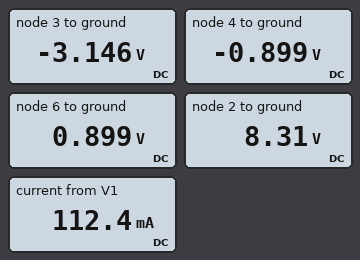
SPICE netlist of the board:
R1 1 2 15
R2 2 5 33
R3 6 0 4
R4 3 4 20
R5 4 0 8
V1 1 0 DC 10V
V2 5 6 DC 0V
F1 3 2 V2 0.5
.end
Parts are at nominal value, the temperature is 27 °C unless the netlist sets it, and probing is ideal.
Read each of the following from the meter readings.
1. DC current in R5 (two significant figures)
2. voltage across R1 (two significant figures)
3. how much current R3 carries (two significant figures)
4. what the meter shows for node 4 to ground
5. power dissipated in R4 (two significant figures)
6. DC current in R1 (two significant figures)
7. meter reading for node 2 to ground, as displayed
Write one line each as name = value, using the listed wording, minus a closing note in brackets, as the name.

DC current in R5 = 110 mA
voltage across R1 = 1.7 V
how much current R3 carries = 220 mA
what the meter shows for node 4 to ground = -0.899 V
power dissipated in R4 = 250 mW
DC current in R1 = 110 mA
meter reading for node 2 to ground, as displayed = 8.31 V
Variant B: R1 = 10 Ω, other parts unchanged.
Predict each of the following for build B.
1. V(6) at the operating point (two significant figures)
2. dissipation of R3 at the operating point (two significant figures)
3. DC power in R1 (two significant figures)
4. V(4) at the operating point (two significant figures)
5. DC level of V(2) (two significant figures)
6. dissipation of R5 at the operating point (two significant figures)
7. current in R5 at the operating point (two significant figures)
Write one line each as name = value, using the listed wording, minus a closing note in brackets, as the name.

V(6) at the operating point = 950 mV
dissipation of R3 at the operating point = 230 mW
DC power in R1 = 140 mW
V(4) at the operating point = -950 mV
DC level of V(2) = 8.8 V
dissipation of R5 at the operating point = 110 mW
current in R5 at the operating point = 120 mA
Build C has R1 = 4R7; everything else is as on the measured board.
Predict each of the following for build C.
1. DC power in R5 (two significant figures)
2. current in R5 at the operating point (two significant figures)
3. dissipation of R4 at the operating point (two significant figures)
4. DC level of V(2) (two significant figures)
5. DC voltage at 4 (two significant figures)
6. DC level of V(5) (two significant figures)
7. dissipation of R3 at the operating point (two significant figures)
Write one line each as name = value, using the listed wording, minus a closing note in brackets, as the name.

DC power in R5 = 130 mW
current in R5 at the operating point = 130 mA
dissipation of R4 at the operating point = 320 mW
DC level of V(2) = 9.4 V
DC voltage at 4 = -1.0 V
DC level of V(5) = 1.0 V
dissipation of R3 at the operating point = 260 mW
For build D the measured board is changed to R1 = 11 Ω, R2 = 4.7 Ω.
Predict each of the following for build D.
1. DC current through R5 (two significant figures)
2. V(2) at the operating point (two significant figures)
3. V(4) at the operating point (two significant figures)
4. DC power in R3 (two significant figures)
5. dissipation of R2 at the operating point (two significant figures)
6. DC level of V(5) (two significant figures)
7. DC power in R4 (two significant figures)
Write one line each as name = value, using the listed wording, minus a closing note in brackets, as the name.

DC current through R5 = 350 mA
V(2) at the operating point = 6.1 V
V(4) at the operating point = -2.8 V
DC power in R3 = 2.0 W
dissipation of R2 at the operating point = 2.3 W
DC level of V(5) = 2.8 V
DC power in R4 = 2.5 W
